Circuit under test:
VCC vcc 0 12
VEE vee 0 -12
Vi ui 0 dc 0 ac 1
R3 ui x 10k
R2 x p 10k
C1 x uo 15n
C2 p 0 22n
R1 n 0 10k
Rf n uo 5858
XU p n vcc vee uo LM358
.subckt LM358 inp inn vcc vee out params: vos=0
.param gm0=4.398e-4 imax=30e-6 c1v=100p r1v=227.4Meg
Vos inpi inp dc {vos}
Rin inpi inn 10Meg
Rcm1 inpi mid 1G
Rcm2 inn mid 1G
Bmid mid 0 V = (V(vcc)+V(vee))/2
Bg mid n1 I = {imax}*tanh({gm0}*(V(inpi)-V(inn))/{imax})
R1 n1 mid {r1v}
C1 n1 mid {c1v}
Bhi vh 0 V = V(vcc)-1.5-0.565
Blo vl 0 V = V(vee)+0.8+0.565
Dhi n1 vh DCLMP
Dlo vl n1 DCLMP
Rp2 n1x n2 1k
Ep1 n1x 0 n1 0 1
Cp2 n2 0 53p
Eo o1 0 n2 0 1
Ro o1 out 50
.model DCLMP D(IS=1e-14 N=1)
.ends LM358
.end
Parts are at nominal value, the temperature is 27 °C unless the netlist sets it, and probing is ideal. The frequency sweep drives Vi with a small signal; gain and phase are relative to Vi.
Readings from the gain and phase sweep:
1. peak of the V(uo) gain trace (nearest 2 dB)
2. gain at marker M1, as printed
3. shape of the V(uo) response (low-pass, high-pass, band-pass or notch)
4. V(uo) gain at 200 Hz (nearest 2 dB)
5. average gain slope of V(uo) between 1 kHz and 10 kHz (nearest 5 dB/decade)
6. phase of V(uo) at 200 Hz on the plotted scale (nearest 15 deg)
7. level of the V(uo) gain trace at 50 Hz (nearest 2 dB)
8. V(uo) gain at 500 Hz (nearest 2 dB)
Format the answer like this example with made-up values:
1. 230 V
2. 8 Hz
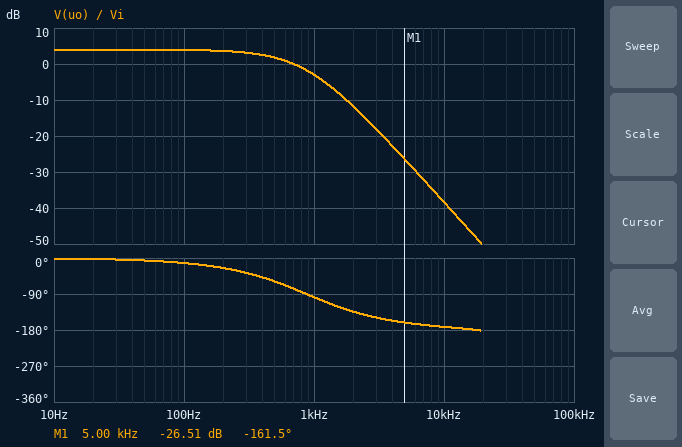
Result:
1. 4 dB
2. -26.51 dB
3. low-pass
4. 4 dB
5. -35 dB/decade
6. -30 deg
7. 4 dB
8. 2 dB
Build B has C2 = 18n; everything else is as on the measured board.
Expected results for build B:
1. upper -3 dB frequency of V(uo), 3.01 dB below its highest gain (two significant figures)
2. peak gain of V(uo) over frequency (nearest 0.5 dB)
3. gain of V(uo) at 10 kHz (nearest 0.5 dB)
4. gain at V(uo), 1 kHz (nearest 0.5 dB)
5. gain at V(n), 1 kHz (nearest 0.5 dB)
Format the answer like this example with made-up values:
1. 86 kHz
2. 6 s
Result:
1. 810 Hz
2. 4.0 dB
3. -36.5 dB
4. -0.5 dB
5. -4.5 dB
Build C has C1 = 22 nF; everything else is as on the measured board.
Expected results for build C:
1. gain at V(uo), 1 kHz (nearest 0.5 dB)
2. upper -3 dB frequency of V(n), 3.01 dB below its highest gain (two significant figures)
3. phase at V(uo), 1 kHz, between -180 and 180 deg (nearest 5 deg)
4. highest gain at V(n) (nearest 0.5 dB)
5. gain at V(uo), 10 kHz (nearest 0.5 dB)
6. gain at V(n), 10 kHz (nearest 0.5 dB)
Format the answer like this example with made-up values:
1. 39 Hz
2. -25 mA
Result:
1. -2.5 dB
2. 720 Hz
3. -115 deg
4. 0 dB
5. -41.5 dB
6. -45.5 dB
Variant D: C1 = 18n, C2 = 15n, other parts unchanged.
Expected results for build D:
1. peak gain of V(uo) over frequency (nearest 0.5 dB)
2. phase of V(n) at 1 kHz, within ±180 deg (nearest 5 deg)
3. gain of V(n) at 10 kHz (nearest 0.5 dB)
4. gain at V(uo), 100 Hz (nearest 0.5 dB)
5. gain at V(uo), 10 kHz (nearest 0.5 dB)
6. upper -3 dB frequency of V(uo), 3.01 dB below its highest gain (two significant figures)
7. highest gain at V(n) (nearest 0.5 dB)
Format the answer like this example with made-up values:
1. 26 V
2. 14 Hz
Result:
1. 4.5 dB
2. -95 deg
3. -40.5 dB
4. 4.0 dB
5. -36.5 dB
6. 1.1 kHz
7. 0.5 dB
